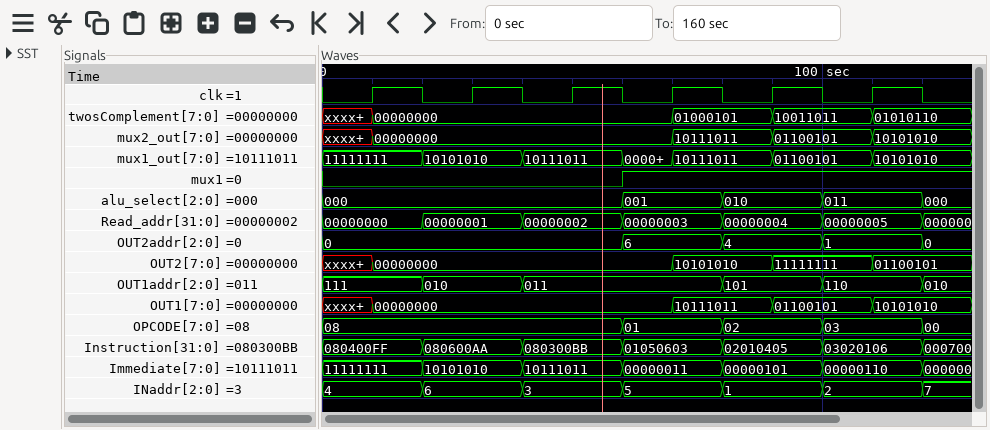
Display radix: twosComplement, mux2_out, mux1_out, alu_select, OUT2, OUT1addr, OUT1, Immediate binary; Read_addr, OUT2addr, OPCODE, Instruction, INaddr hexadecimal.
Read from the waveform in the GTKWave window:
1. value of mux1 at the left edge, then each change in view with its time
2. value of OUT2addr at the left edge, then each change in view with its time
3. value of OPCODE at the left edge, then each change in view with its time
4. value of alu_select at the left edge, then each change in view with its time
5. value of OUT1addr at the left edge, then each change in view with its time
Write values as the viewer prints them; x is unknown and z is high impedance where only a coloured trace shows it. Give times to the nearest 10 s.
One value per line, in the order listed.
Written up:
0, 1 at 60 s
0, 6 at 60 s, 4 at 80 s, 1 at 100 s, 0 at 120 s
08, 01 at 60 s, 02 at 80 s, 03 at 100 s, 00 at 120 s
000, 001 at 60 s, 010 at 80 s, 011 at 100 s, 000 at 120 s
111, 010 at 20 s, 011 at 40 s, 101 at 80 s, 110 at 100 s, 010 at 120 s
